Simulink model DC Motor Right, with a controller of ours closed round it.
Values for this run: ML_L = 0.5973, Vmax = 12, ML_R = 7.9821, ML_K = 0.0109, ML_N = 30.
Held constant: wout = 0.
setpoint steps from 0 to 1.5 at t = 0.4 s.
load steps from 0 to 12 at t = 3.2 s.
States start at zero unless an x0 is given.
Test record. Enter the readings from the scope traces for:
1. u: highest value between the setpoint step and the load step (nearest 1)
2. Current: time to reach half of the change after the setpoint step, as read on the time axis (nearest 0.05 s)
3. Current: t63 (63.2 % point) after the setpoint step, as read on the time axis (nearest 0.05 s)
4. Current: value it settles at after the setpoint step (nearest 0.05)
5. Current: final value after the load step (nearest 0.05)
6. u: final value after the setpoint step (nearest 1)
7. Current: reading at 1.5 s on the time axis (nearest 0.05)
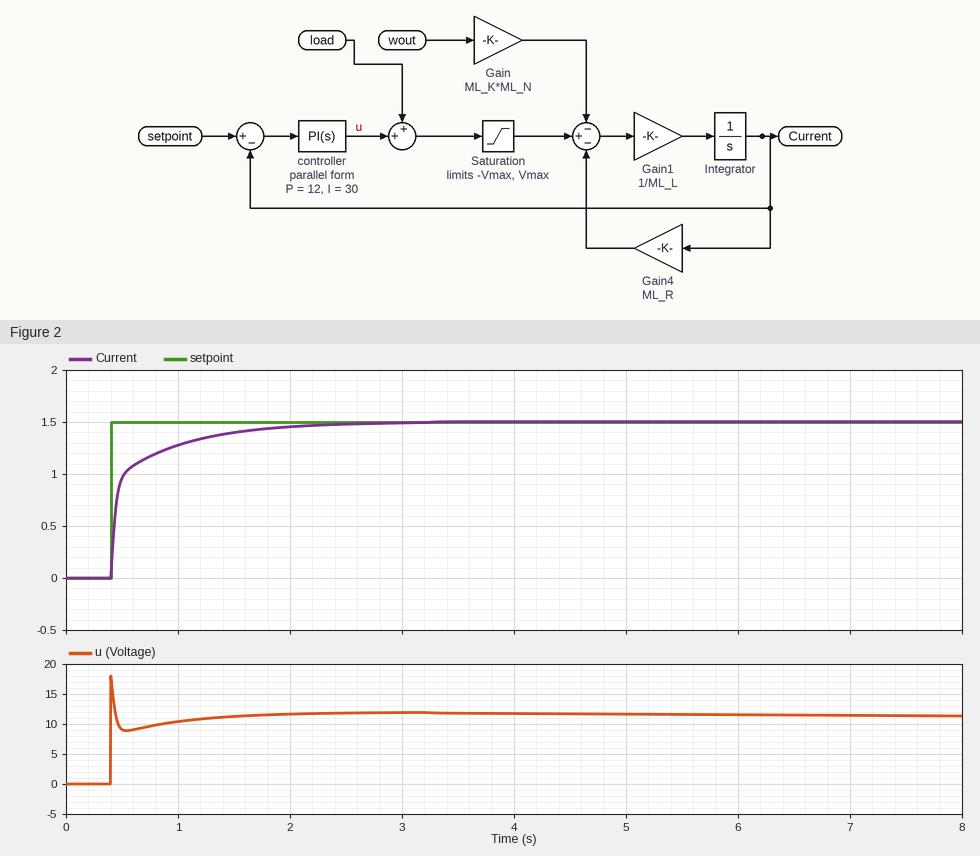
18
0.45 s
0.50 s
1.50
1.50
12
1.40
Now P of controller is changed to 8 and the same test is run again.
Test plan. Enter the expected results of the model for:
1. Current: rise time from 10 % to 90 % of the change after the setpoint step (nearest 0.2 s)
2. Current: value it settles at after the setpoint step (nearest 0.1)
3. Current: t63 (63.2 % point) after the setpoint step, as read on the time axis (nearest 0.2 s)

0.8 s
1.5
0.6 s
